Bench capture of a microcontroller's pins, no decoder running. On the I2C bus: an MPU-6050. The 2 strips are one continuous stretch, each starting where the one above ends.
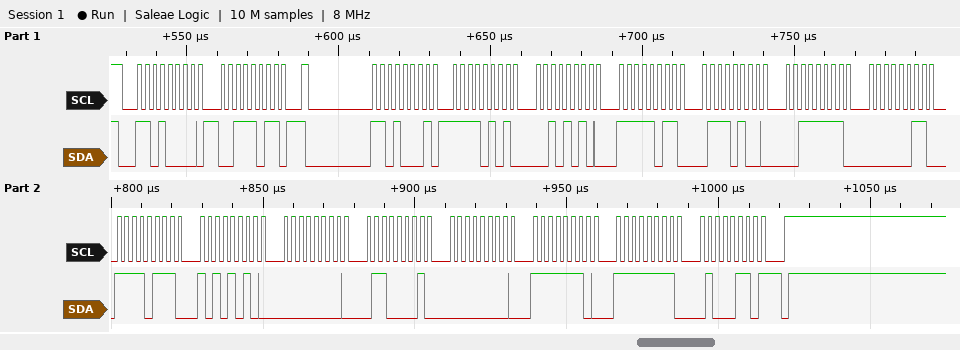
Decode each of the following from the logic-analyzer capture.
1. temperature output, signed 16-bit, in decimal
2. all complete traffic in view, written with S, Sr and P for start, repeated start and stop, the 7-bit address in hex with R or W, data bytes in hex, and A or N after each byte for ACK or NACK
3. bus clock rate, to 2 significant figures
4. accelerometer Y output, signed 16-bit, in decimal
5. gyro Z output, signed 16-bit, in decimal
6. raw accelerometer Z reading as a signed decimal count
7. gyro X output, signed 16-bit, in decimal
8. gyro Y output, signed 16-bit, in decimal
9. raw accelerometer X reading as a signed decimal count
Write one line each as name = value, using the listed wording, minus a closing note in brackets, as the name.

temperature output, signed 16-bit, in decimal = -2134
all complete traffic in view, written with S, Sr and P for start, repeated start and stop, the 7-bit address in hex with R or W, data bytes in hex, and A or N after each byte for ACK or NACK = S 68W A 3B A Sr 68R A F5 A 2A A FB A 74 A 3F A 03 A F7 A AA A 00 A 61 A 00 A FE A FF A 46 N P
bus clock rate, to 2 significant figures = 400 kHz
accelerometer Y output, signed 16-bit, in decimal = -1164
gyro Z output, signed 16-bit, in decimal = -186
raw accelerometer Z reading as a signed decimal count = 16131
gyro X output, signed 16-bit, in decimal = 97
gyro Y output, signed 16-bit, in decimal = 254
raw accelerometer X reading as a signed decimal count = -2774
